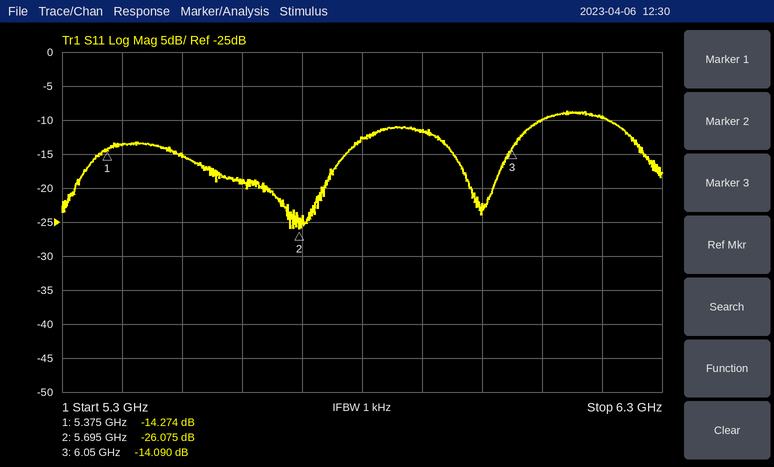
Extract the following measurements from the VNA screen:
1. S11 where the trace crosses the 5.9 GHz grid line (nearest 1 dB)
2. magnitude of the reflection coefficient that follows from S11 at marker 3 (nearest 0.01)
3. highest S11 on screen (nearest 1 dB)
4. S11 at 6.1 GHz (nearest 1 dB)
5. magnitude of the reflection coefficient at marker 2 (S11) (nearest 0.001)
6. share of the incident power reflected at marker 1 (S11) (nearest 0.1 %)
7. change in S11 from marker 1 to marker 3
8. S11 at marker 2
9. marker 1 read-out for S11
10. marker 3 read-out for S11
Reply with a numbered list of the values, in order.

1. -12 dB
2. 0.20
3. -9 dB
4. -10 dB
5. 0.050
6. 3.7 %
7. 0.184 dB
8. -26.075 dB
9. -14.274 dB
10. -14.090 dB
